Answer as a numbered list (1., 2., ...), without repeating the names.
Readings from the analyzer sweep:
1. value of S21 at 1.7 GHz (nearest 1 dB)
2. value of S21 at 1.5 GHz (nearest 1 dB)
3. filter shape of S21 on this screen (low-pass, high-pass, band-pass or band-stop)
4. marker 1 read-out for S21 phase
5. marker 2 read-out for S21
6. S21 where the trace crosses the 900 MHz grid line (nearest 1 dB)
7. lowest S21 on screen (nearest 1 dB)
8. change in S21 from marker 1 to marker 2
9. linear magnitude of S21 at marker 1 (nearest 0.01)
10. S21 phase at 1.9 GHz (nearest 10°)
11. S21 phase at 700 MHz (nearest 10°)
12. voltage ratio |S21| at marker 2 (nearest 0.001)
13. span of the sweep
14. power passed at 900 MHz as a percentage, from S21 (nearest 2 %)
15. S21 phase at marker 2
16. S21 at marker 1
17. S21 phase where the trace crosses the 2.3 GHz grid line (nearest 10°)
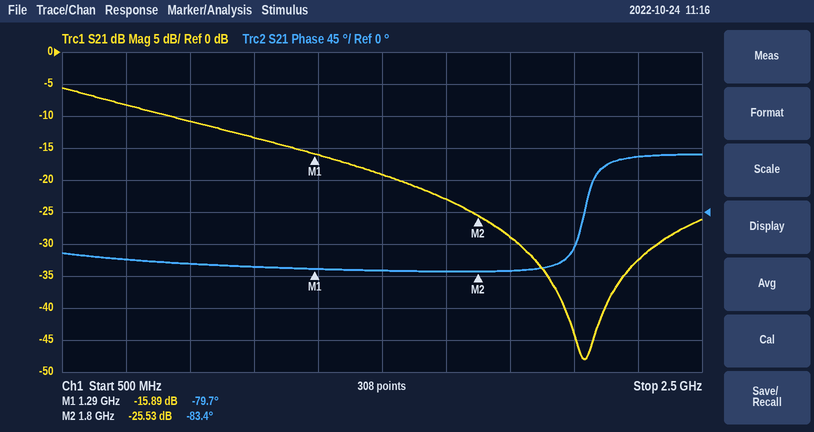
1. -23 dB
2. -19 dB
3. low-pass
4. -79.7°
5. -25.53 dB
6. -11 dB
7. -48 dB
8. -9.64 dB
9. 0.16
10. -80°
11. -70°
12. 0.053
13. 2 GHz
14. 8 %
15. -83.4°
16. -15.89 dB
17. 80°
